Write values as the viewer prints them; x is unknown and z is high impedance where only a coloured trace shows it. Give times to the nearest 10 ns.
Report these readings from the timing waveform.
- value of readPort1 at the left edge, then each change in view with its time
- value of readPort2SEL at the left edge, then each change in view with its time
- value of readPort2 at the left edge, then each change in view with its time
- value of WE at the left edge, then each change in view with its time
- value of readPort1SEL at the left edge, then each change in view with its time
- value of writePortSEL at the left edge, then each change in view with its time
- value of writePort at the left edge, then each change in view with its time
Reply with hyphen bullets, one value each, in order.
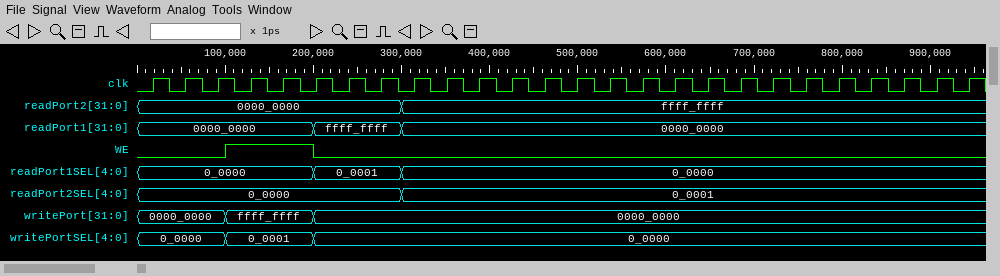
- 0000_0000, ffff_ffff at 200 ns, 0000_0000 at 300 ns
- 0_0000, 0_0001 at 300 ns
- 0000_0000, ffff_ffff at 300 ns
- 0, 1 at 100 ns, 0 at 200 ns
- 0_0000, 0_0001 at 200 ns, 0_0000 at 300 ns
- 0_0000, 0_0001 at 100 ns, 0_0000 at 200 ns
- 0000_0000, ffff_ffff at 100 ns, 0000_0000 at 200 ns
